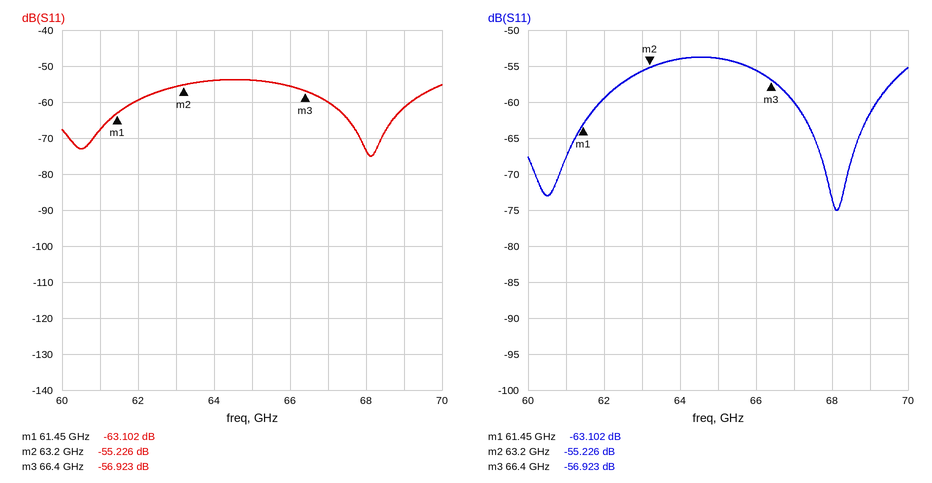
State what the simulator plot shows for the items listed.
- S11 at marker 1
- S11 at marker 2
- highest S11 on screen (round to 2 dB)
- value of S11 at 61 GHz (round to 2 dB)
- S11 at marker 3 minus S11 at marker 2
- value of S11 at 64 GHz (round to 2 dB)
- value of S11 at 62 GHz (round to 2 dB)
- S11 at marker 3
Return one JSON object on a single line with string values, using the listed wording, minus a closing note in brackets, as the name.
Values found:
{"S11 at marker 1": "-63.102 dB", "S11 at marker 2": "-55.226 dB", "highest S11 on screen": "-54 dB", "value of S11 at 61 GHz": "-68 dB", "S11 at marker 3 minus S11 at marker 2": "-1.697 dB", "value of S11 at 64 GHz": "-54 dB", "value of S11 at 62 GHz": "-60 dB", "S11 at marker 3": "-56.923 dB"}
